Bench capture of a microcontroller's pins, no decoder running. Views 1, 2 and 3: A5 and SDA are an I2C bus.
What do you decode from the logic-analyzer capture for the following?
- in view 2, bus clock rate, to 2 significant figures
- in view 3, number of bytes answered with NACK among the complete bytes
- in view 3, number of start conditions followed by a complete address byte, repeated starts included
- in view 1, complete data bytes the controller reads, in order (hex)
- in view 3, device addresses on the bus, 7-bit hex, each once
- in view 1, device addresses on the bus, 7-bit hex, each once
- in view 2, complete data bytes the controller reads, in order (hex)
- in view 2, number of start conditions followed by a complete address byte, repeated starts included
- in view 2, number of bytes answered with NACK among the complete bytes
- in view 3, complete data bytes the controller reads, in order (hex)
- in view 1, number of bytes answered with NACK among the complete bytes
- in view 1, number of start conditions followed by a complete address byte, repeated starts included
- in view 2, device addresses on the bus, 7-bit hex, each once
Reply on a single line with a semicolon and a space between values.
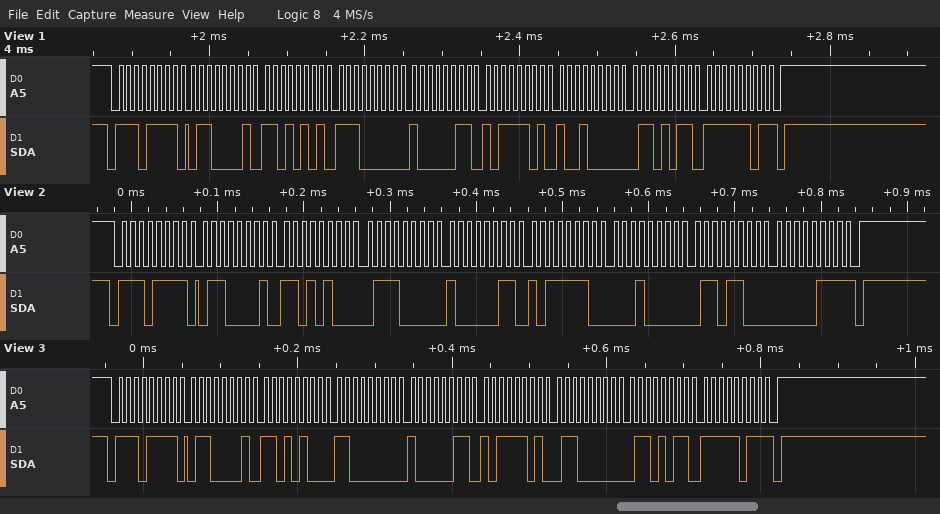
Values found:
100 kHz; 1; 1; 61 D5 E0 83 BD 90 6B FD; 0x77; 0x77; 61 D4 70 83 BE 10 6C 07; 1; 1; 61 D4 C0 83 BD 60 6B FB; 1; 1; 0x77
